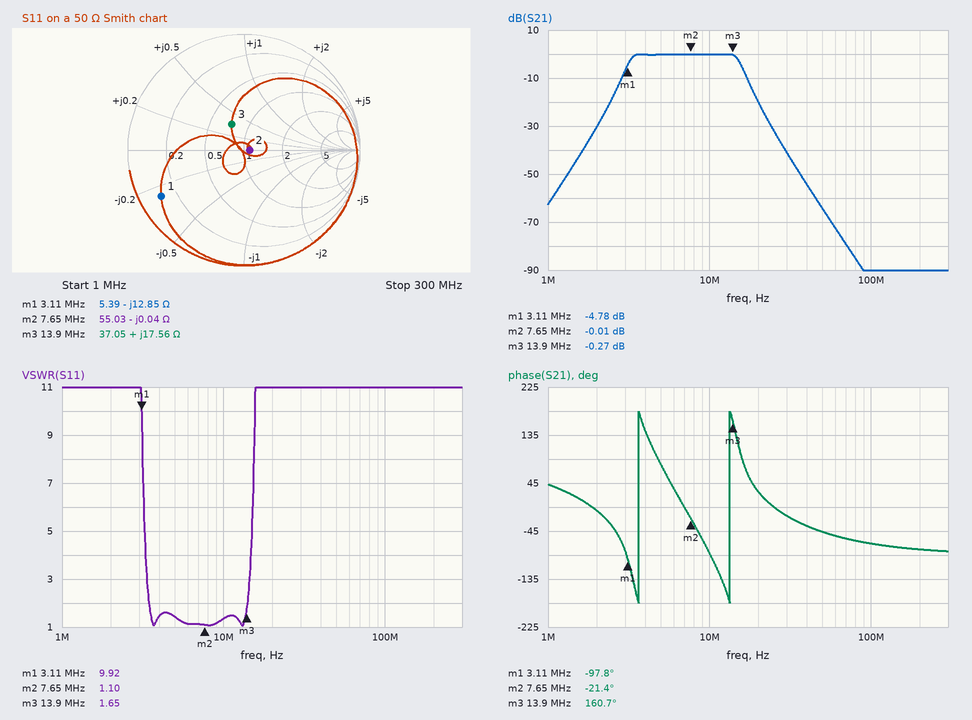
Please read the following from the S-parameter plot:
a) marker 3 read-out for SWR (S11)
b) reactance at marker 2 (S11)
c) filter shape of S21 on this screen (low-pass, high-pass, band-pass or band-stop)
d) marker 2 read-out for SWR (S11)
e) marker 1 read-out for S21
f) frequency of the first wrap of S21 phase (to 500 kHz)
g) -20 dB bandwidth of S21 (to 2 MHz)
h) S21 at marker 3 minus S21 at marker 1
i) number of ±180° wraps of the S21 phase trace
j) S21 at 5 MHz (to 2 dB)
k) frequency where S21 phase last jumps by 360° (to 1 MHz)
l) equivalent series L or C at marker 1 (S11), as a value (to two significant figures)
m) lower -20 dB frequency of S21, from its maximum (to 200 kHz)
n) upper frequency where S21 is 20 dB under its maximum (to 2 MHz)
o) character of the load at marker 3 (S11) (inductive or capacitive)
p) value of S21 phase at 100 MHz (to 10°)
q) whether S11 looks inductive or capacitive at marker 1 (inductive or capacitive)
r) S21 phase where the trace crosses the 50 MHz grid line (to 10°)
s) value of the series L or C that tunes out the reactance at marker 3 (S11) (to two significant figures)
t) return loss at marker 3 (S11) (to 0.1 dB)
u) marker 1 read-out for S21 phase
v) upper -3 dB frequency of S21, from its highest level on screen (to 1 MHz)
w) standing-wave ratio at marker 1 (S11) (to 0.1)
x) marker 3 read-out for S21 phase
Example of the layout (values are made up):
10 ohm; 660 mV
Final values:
1.65; -0.04 Ω; band-pass; 1.10; -4.78 dB; 3.5 MHz; 18 MHz; 4.51 dB; 2; 0 dB; 13 MHz; 4.0 nF; 2.4 MHz; 20 MHz; inductive; -70°; capacitive; -50°; 650 pF; 12.2 dB; -97.8°; 15 MHz; 9.9; 160.7°
